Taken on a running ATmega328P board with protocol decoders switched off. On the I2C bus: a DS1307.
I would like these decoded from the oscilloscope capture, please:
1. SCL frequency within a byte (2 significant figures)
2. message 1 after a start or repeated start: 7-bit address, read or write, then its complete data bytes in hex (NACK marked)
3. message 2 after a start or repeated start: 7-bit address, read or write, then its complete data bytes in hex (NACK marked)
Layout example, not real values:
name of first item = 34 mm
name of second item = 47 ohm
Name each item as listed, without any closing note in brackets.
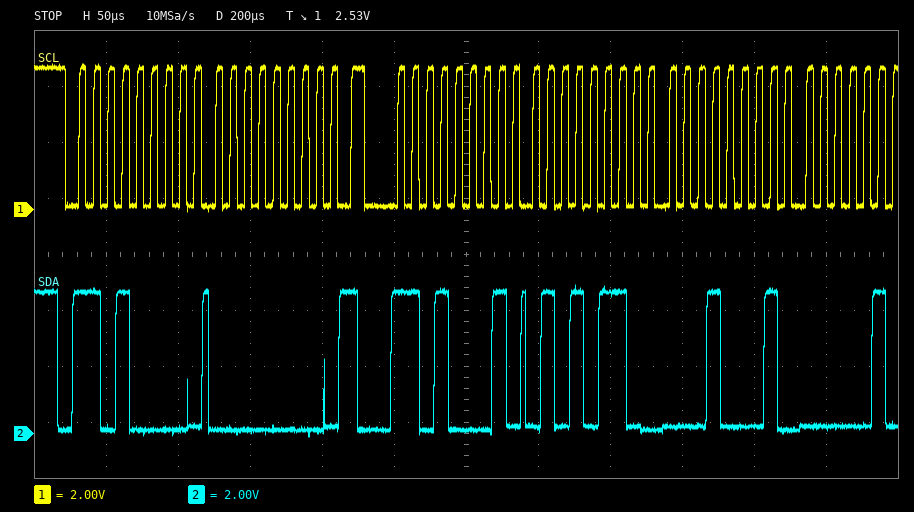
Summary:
SCL frequency within a byte = 100 kHz
message 1 after a start or repeated start: 7-bit address, read or write, then its complete data bytes in hex = 0x68 write: 00
message 2 after a start or repeated start: 7-bit address, read or write, then its complete data bytes in hex = 0x68 read: 56 11
